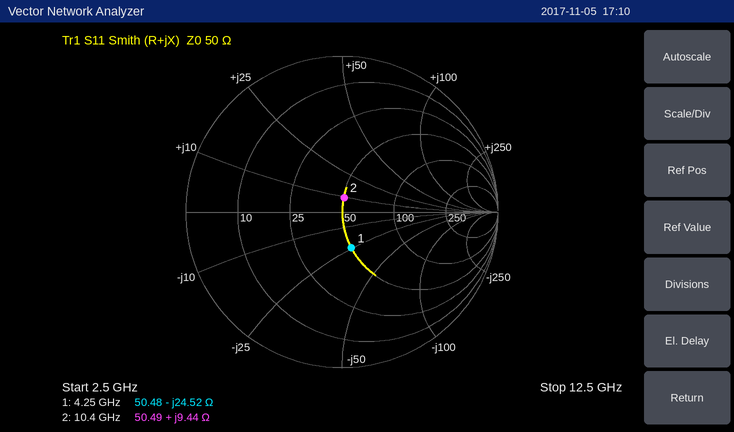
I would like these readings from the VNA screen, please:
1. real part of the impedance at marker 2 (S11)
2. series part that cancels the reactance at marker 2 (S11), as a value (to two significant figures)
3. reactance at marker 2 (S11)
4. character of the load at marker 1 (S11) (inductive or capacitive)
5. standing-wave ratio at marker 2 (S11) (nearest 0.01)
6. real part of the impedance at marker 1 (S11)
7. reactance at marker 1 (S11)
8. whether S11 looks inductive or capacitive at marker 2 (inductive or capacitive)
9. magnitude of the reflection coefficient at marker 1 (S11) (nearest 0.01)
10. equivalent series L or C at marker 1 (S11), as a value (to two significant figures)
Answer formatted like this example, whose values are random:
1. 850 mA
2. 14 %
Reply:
1. 50.49 Ω
2. 1.6 pF
3. +9.44 Ω
4. capacitive
5. 1.21
6. 50.48 Ω
7. -24.52 Ω
8. inductive
9. 0.24
10. 1.5 pF
